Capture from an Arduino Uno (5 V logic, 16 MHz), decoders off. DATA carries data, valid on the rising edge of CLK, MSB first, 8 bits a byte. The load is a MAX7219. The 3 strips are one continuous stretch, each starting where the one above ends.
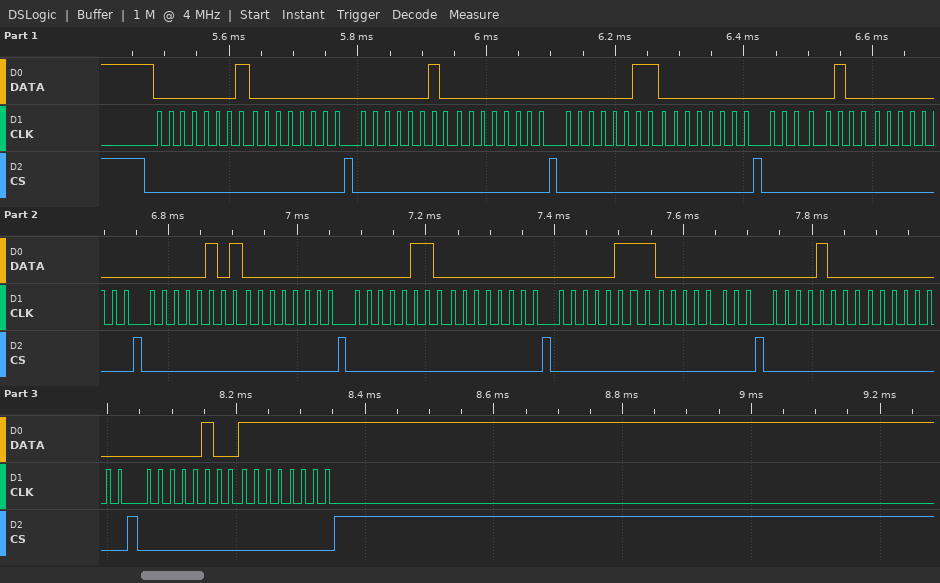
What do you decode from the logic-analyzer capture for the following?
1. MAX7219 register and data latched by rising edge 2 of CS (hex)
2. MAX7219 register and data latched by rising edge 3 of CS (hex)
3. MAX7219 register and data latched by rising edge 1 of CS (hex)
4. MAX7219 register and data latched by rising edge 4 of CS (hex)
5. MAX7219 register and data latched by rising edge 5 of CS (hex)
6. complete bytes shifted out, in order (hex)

register 0x2, data 0x00
register 0x3, data 0x00
register 0x1, data 0x00
register 0x4, data 0x00
register 0x5, data 0x00
01 00 02 00 03 00 04 00 05 00 06 00 07 00 08 00 04 FF
